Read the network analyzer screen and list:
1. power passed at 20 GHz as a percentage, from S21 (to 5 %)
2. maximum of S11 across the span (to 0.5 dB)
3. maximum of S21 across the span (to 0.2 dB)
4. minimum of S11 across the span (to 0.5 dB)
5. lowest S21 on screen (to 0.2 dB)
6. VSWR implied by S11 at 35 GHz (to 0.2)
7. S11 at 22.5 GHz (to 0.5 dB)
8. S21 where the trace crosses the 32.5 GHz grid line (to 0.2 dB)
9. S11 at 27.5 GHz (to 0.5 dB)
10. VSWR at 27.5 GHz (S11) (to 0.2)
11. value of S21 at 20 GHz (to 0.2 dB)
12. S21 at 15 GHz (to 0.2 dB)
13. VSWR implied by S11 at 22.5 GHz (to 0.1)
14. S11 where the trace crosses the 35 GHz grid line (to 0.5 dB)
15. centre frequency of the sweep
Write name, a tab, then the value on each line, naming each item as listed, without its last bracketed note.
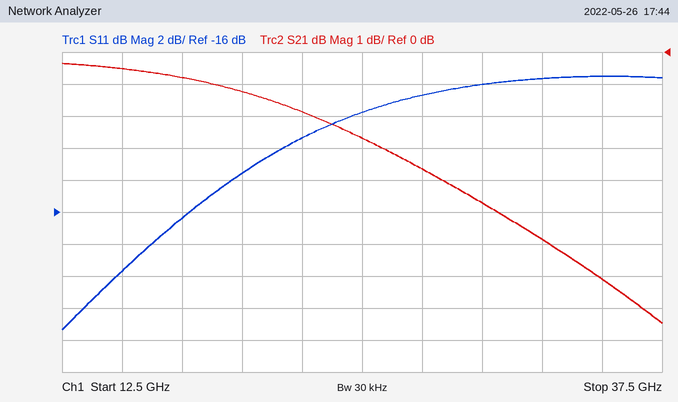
power passed at 20 GHz as a percentage, from S21	75 %
maximum of S11 across the span	-7.5 dB
maximum of S21 across the span	-0.4 dB
minimum of S11 across the span	-23.5 dB
lowest S21 on screen	-8.4 dB
VSWR implied by S11 at 35 GHz	2.4
S11 at 22.5 GHz	-11.5 dB
S21 where the trace crosses the 32.5 GHz grid line	-5.8 dB
S11 at 27.5 GHz	-8.5 dB
VSWR at 27.5 GHz (S11)	2.2
value of S21 at 20 GHz	-1.2 dB
S21 at 15 GHz	-0.6 dB
VSWR implied by S11 at 22.5 GHz	1.7
S11 where the trace crosses the 35 GHz grid line	-7.5 dB
centre frequency of the sweep	25 GHz
